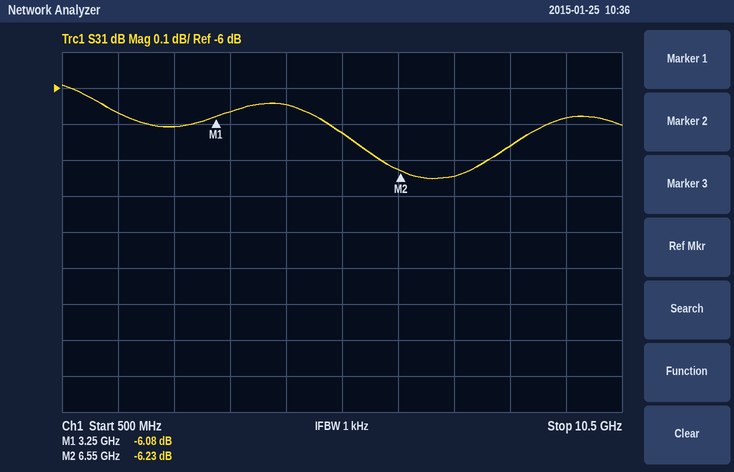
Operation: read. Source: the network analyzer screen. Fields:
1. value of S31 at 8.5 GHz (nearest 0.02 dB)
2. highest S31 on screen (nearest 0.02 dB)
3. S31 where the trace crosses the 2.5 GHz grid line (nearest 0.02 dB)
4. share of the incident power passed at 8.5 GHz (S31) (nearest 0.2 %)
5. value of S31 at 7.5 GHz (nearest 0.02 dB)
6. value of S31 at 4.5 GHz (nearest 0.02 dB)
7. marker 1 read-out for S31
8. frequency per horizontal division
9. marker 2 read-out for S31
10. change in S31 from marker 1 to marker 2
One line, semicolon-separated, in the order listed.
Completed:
-6.16 dB; -6.00 dB; -6.10 dB; 24.2 %; -6.24 dB; -6.04 dB; -6.08 dB; 1 GHz; -6.23 dB; -0.15 dB
